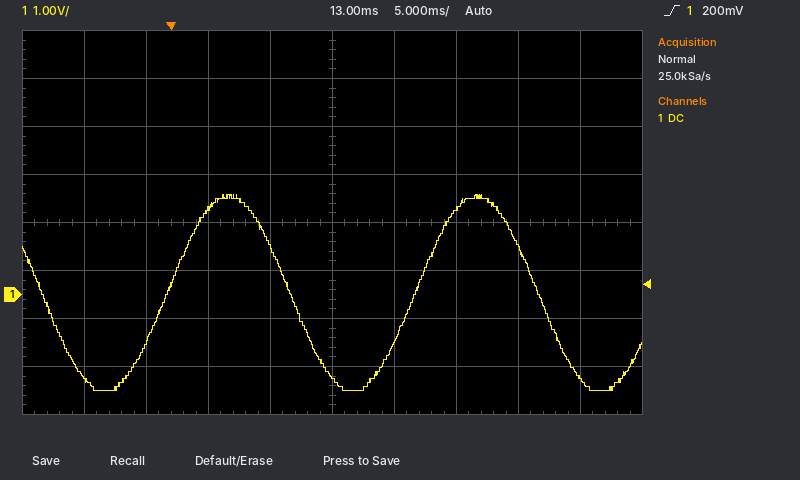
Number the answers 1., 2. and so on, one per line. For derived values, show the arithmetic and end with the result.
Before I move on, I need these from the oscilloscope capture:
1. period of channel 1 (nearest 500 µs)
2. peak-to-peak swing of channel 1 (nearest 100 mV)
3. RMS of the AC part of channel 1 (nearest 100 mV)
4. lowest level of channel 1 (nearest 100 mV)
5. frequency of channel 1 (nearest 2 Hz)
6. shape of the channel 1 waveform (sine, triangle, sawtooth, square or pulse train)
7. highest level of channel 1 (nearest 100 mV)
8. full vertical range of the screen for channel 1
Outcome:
1. 20.0 ms
2. 2.1 V − (-2.0 V) = 4.1 V
3. 4.1 V / (2√2) ≈ 1.4 V
4. -2.0 V
5. 1 / 20.0 ms ≈ 50 Hz
6. sine
7. 2.1 V
8. 8 V
